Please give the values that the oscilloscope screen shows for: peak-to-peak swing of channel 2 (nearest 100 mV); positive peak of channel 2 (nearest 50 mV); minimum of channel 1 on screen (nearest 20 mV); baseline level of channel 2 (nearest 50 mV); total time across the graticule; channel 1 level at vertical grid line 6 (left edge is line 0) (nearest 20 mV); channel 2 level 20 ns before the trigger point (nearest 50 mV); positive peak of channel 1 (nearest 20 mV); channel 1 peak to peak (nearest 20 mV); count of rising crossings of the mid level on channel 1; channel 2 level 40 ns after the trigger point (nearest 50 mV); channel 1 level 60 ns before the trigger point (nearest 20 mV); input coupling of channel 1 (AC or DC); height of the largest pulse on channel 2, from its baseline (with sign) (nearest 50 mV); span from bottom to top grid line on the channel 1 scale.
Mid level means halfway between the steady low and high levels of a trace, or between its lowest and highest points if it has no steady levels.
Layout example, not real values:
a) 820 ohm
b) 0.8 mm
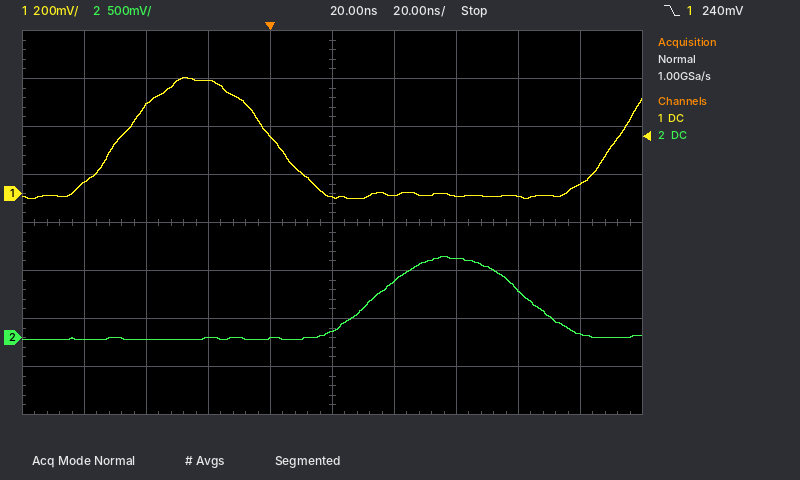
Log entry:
a) 900 mV
b) 850 mV
c) -20 mV
d) 0 mV
e) 200 ns
f) 0 mV
g) 0 mV
h) 480 mV
i) 500 mV
j) 2
k) 600 mV
l) 40 mV
m) DC
n) +850 mV
o) 1.6 V
